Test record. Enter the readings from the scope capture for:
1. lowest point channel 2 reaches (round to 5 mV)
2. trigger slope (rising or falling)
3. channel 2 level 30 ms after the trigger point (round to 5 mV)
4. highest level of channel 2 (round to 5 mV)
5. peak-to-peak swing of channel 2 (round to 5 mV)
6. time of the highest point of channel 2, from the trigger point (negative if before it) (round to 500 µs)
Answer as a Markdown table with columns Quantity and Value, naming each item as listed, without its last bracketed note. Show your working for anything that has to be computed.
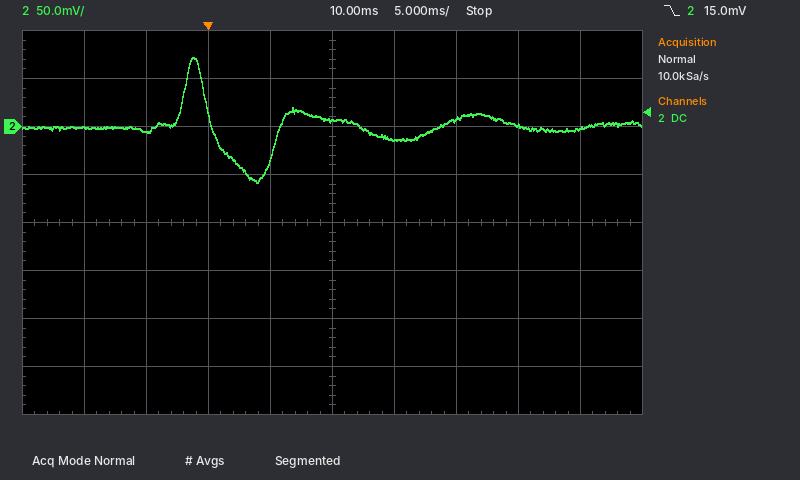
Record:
| Quantity | Value |
|---|---|
| lowest point channel 2 reaches | -60 mV |
| trigger slope | falling |
| channel 2 level 30 ms after the trigger point | 0 mV |
| highest level of channel 2 | 70 mV |
| peak-to-peak swing of channel 2 | 70 mV − (-60 mV) = 130 mV |
| time of the highest point of channel 2, from the trigger point (negative if before it) | -1.0 ms |
